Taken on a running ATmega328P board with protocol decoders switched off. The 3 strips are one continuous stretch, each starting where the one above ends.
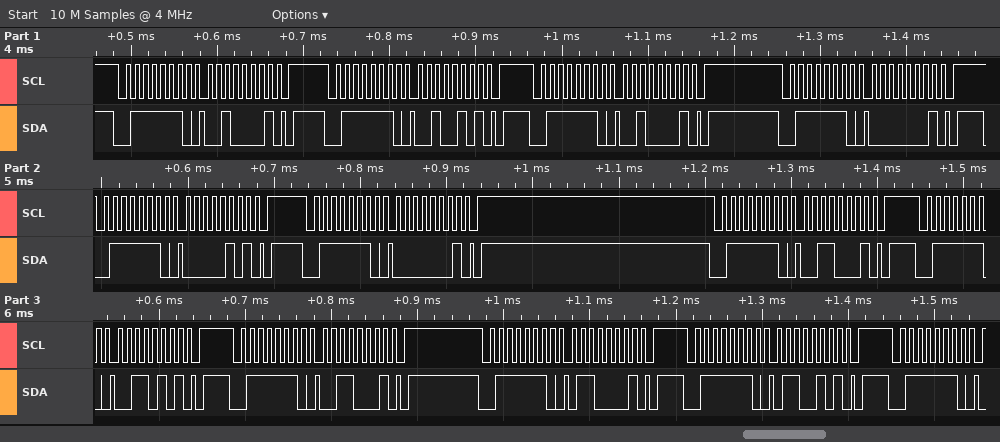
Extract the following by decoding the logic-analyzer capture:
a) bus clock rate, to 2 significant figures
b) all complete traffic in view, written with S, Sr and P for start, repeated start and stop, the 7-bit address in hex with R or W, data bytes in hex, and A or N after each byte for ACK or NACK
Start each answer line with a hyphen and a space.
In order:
- 100 kHz
- S 3FW A 21 A P S 3FW A 25 A P S 3FW A 21 A P S 3FW A 01 A P S 3FW A 05 A P S 3FW A 01 A P S 3FW A 31 A P S 3FW A 35 A P S 3FW A 31 A P S 3FW A 61 A P S 3FW A 65 A P S 3FW A
